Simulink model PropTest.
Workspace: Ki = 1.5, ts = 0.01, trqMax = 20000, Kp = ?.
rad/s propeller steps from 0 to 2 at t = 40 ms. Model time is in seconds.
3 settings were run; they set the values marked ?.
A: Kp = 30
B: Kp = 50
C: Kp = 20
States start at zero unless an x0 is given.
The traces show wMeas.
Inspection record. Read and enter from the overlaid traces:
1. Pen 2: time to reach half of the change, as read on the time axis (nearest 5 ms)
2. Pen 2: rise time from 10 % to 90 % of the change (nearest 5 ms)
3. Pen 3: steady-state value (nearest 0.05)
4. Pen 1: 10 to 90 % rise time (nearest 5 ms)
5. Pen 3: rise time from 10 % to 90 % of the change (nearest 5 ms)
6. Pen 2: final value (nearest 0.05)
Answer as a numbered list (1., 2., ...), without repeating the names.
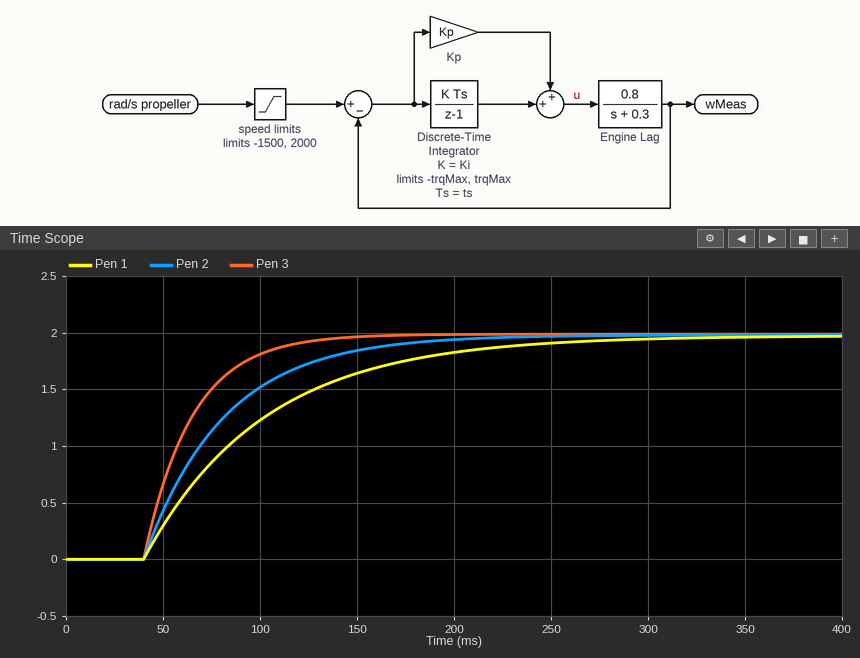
1. 70 ms
2. 90 ms
3. 2.00
4. 135 ms
5. 55 ms
6. 2.00
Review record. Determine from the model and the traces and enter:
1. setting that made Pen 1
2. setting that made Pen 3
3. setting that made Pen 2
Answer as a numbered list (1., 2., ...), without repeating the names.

1. C
2. B
3. A
